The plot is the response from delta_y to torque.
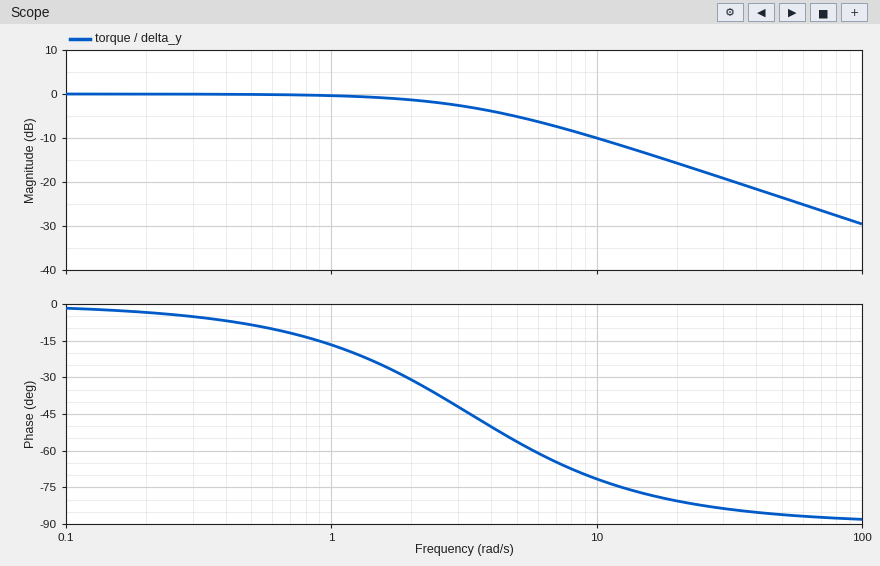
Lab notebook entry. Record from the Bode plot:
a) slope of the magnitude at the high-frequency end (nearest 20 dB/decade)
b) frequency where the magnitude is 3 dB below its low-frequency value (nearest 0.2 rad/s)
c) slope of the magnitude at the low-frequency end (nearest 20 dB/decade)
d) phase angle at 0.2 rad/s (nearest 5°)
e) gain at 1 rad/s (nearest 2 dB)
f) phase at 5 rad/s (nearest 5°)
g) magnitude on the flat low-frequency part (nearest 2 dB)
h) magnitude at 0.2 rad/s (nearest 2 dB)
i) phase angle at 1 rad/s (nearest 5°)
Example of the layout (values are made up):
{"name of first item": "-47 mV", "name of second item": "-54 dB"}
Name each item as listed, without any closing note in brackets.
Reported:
{"slope of the magnitude at the high-frequency end": "-20 dB/decade", "frequency where the magnitude is 3 dB below its low-frequency value": "3.4 rad/s", "slope of the magnitude at the low-frequency end": "0 dB/decade", "phase angle at 0.2 rad/s": "-5°", "gain at 1 rad/s": "0 dB", "phase at 5 rad/s": "-55°", "magnitude on the flat low-frequency part": "0 dB", "magnitude at 0.2 rad/s": "0 dB", "phase angle at 1 rad/s": "-15°"}
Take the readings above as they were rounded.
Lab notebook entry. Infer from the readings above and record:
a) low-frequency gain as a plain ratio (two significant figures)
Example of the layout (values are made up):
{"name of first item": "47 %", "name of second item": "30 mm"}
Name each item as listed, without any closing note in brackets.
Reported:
{"low-frequency gain as a plain ratio": "1.0"}
